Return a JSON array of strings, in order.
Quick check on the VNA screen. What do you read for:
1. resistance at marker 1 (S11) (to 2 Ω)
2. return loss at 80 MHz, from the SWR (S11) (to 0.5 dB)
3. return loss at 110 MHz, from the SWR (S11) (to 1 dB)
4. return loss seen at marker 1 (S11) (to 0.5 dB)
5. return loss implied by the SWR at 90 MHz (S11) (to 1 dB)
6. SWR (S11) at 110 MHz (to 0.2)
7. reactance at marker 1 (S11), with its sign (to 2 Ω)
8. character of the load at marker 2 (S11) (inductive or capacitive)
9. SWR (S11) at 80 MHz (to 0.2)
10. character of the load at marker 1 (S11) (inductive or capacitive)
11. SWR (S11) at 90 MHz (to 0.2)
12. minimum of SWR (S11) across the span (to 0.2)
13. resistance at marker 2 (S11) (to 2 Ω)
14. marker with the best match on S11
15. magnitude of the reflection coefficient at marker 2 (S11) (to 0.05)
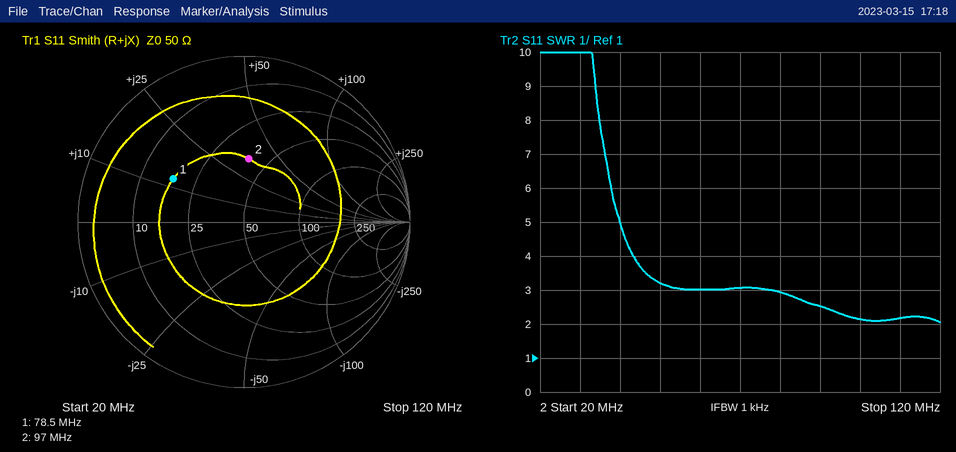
["18 Ω", "6.0 dB", "9 dB", "6.0 dB", "7 dB", "2.2", "+12 Ω", "inductive", "3.0", "inductive", "2.6", "2.0", "40 Ω", "marker 2", "0.40"]
